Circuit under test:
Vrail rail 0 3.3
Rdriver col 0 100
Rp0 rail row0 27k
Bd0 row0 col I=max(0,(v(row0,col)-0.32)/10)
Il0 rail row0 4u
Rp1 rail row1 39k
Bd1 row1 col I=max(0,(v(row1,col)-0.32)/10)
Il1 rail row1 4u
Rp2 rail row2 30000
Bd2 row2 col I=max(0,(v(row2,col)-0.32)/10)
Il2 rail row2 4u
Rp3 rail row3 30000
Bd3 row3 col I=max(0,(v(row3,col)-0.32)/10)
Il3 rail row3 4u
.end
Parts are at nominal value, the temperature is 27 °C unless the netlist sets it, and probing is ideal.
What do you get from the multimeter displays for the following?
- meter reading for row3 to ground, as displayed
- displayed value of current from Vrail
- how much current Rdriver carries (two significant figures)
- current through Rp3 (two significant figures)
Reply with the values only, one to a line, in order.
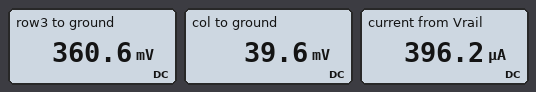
360.6 mV
396.2 µA
400 µA
98 µA
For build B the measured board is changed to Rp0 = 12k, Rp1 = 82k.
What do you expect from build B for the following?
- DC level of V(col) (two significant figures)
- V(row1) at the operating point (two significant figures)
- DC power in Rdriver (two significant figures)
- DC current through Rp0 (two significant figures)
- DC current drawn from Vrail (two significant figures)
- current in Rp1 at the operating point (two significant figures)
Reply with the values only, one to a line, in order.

49 mV
370 mV
24 µW
240 µA
490 µA
36 µA
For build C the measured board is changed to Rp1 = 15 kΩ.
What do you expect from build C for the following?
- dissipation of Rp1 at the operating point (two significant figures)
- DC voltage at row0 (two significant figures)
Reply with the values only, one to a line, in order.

570 µW
370 mV
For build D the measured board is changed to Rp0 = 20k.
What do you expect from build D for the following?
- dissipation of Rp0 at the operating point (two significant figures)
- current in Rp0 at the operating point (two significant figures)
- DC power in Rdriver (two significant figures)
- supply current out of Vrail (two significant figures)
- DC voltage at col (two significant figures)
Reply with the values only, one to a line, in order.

430 µW
150 µA
19 µW
430 µA
43 mV
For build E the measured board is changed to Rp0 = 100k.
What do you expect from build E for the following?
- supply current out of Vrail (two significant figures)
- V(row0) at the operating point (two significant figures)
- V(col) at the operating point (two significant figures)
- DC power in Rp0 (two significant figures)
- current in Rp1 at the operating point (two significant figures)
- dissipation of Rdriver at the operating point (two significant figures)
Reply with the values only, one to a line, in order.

320 µA
350 mV
32 mV
87 µW
76 µA
10 µW
